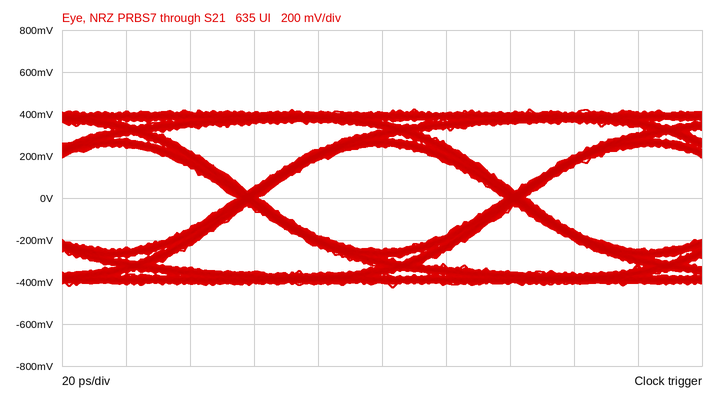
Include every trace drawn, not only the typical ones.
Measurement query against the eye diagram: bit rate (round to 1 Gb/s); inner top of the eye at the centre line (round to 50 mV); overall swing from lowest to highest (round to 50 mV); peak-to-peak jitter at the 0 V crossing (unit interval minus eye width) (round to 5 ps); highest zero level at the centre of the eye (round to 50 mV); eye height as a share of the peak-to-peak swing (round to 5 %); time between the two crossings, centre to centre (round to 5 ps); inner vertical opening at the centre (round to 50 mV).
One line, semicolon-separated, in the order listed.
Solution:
12 Gb/s; 250 mV; 850 mV; 5 ps; -250 mV; 60 %; 85 ps; 500 mV
